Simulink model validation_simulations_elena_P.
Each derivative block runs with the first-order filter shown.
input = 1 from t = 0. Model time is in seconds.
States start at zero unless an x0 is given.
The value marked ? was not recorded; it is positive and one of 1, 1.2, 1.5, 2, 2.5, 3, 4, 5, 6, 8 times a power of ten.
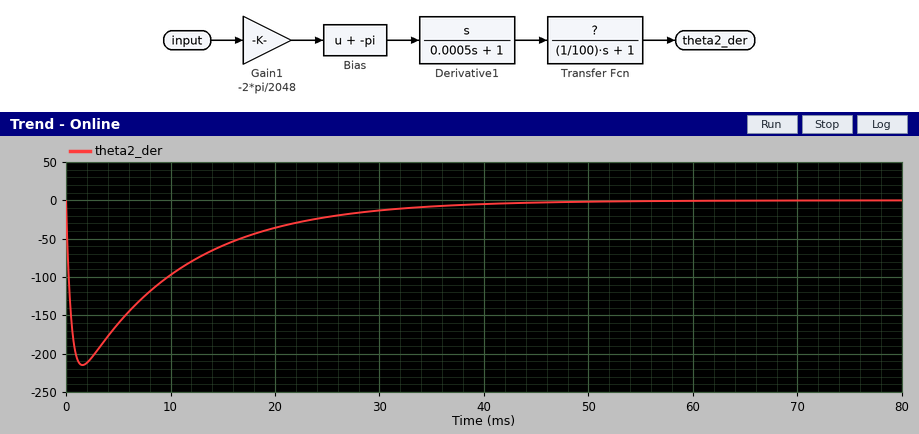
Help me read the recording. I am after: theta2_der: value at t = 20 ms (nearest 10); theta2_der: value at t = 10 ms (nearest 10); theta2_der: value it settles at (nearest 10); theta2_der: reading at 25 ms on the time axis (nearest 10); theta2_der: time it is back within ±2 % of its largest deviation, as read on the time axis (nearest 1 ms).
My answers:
-40
-100
0
-20
41 ms
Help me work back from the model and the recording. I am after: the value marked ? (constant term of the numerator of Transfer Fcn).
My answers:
0.8
